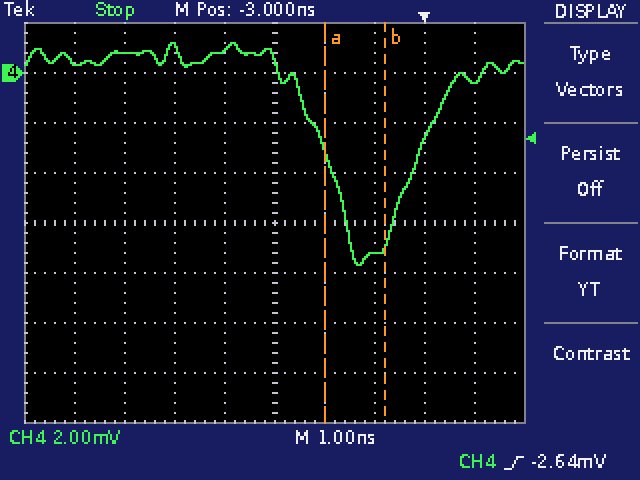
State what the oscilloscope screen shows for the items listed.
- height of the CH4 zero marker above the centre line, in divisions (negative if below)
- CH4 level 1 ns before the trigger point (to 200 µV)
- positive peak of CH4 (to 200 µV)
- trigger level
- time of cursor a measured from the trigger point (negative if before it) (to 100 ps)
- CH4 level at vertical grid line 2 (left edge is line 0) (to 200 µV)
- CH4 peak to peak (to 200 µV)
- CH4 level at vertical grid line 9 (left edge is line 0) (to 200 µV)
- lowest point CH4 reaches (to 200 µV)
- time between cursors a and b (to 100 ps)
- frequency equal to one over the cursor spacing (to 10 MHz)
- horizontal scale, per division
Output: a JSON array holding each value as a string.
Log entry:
["+3.0 div", "-7.2 mV", "1.2 mV", "-2.64 mV", "-2.0 ns", "800 µV", "8.8 mV", "-400 µV", "-7.6 mV", "1.2 ns", "830 MHz", "1 ns"]
